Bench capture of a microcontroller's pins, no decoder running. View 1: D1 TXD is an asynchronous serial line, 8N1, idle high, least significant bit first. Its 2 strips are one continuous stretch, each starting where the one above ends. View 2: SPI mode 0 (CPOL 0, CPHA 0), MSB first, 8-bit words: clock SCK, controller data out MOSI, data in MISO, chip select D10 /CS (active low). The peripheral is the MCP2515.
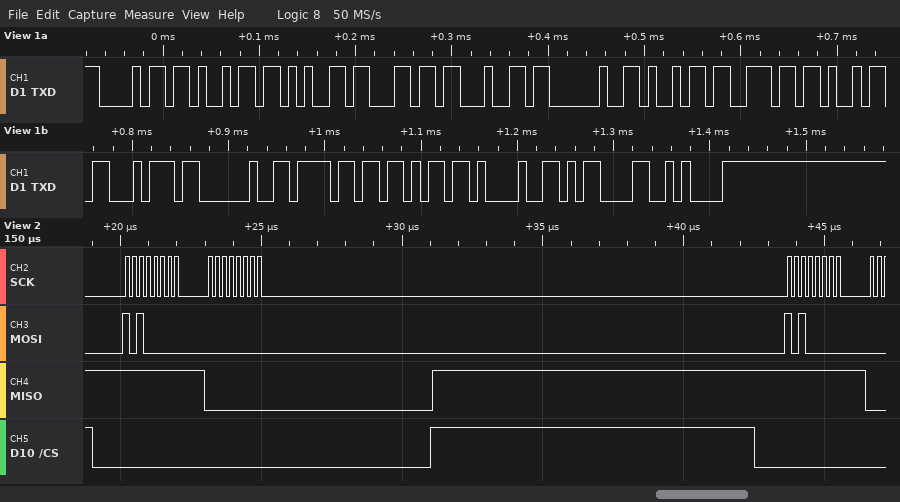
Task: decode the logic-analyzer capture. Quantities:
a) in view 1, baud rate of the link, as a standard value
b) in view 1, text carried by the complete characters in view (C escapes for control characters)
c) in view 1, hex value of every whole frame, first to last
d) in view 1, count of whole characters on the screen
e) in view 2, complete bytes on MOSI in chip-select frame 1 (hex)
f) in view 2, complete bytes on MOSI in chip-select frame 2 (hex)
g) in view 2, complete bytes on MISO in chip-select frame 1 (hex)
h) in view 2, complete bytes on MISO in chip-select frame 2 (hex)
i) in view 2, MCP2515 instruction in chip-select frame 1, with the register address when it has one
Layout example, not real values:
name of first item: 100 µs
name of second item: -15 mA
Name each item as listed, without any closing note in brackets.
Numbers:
in view 1, baud rate of the link, as a standard value: 115200 baud
in view 1, text carried by the complete characters in view: "hield init ok!\r\n"
in view 1, hex value of every whole frame, first to last: 68 69 65 6C 64 20 69 6E 69 74 20 6F 6B 21 0D 0A
in view 1, count of whole characters on the screen: 16
in view 2, complete bytes on MOSI in chip-select frame 1: A0 00
in view 2, complete bytes on MOSI in chip-select frame 2: A0
in view 2, complete bytes on MISO in chip-select frame 1: FF 00
in view 2, complete bytes on MISO in chip-select frame 2: FF
in view 2, MCP2515 instruction in chip-select frame 1, with the register address when it has one: READ STATUS
